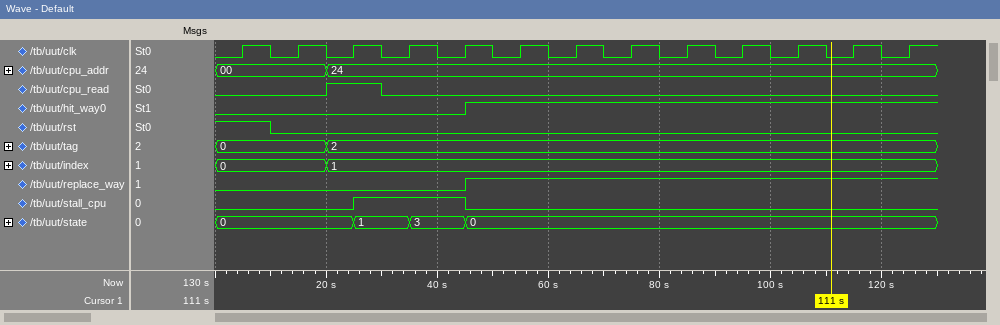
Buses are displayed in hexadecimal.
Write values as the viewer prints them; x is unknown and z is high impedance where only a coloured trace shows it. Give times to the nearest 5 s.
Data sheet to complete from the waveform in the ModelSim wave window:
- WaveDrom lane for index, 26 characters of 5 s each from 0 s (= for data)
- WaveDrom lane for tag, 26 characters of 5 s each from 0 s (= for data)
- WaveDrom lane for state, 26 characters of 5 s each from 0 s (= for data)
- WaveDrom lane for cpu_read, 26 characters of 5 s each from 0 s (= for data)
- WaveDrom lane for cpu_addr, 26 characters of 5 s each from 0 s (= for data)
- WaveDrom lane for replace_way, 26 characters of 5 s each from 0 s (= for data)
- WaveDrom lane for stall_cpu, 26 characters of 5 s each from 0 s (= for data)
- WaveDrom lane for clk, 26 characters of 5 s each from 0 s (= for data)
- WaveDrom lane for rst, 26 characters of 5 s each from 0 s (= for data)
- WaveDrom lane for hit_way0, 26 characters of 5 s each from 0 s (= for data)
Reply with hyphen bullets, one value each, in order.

- {name: 'index', wave: '=...=.....................', data: '0 1'}
- {name: 'tag', wave: '=...=.....................', data: '0 2'}
- {name: 'state', wave: '=....=.=.=................', data: '0 1 3 0'}
- {name: 'cpu_read', wave: '0...1.0...................'}
- {name: 'cpu_addr', wave: '=...=.....................', data: '00 24'}
- {name: 'replace_way', wave: '0........1................'}
- {name: 'stall_cpu', wave: '0....1...0................'}
- {name: 'clk', wave: '01010101010101010101010101'}
- {name: 'rst', wave: '1.0.......................'}
- {name: 'hit_way0', wave: '0........1................'}
